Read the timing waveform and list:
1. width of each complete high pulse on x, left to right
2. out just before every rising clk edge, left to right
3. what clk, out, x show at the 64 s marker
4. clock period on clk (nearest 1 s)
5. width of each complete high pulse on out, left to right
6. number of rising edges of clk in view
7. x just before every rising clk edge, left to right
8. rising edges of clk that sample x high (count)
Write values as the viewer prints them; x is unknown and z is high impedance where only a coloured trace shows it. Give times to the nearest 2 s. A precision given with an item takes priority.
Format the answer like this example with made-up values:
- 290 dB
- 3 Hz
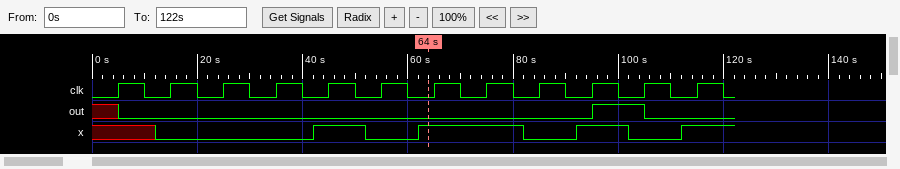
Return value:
- 10 s, 20 s, 10 s
- x 0 0 0 0 0 0 0 0 0 1 0
- clk=0, out=0, x=1
- 10 s
- 10 s
- 12
- x 0 0 0 1 0 1 1 0 1 0 1
- 5
